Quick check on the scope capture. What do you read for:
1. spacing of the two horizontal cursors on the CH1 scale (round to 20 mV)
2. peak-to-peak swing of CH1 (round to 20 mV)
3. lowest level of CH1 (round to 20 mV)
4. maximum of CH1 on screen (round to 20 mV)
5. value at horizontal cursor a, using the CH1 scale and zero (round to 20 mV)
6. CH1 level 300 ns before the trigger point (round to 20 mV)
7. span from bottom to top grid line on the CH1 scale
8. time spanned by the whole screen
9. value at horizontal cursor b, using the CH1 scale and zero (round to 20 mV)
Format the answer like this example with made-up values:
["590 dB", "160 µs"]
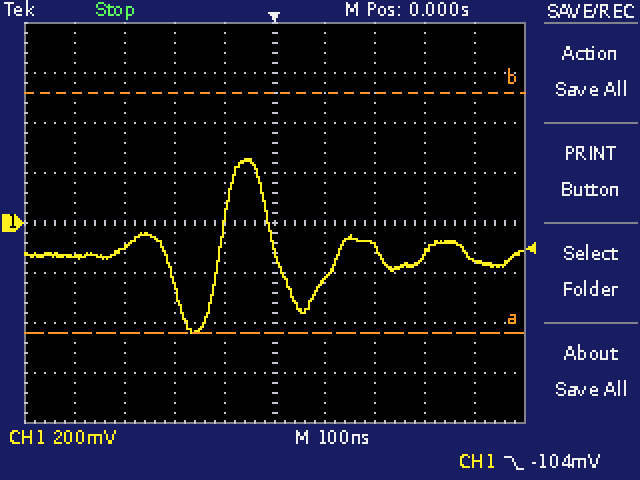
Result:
["960 mV", "700 mV", "-440 mV", "260 mV", "-440 mV", "-100 mV", "1.6 V", "1 µs", "520 mV"]
